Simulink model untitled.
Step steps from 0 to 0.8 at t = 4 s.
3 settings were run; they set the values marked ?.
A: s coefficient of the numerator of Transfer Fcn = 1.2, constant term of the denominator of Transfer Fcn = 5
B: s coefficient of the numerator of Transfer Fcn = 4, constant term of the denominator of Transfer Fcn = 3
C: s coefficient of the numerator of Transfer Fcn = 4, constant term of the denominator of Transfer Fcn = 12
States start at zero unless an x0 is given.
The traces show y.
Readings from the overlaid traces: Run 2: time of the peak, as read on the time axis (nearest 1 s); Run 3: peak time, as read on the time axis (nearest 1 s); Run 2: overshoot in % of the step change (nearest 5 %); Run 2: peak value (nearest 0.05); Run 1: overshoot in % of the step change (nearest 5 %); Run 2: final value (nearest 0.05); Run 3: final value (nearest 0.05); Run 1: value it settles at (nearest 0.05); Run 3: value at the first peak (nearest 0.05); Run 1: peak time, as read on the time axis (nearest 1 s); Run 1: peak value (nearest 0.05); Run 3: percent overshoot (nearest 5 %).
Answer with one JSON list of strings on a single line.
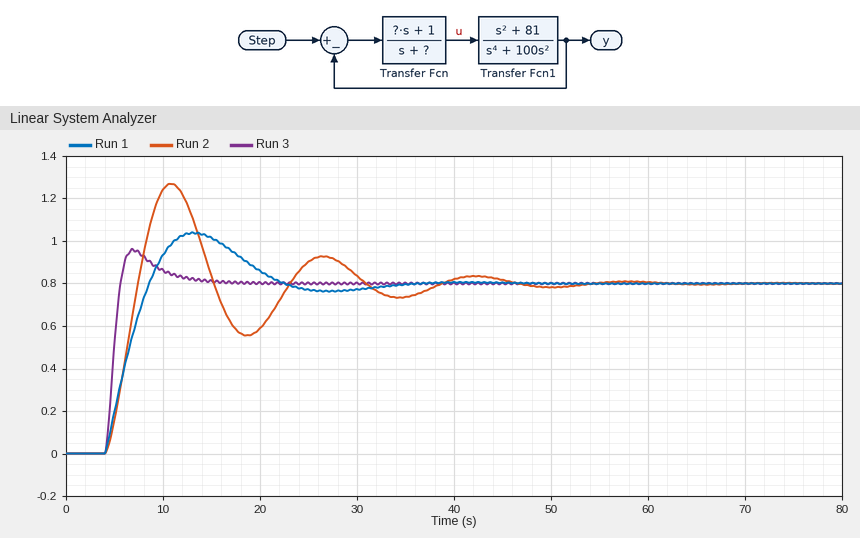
["11 s", "7 s", "60 %", "1.25", "30 %", "0.80", "0.80", "0.80", "0.95", "13 s", "1.05", "20 %"]
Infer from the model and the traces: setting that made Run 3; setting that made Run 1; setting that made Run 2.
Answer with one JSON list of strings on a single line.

["B", "C", "A"]
